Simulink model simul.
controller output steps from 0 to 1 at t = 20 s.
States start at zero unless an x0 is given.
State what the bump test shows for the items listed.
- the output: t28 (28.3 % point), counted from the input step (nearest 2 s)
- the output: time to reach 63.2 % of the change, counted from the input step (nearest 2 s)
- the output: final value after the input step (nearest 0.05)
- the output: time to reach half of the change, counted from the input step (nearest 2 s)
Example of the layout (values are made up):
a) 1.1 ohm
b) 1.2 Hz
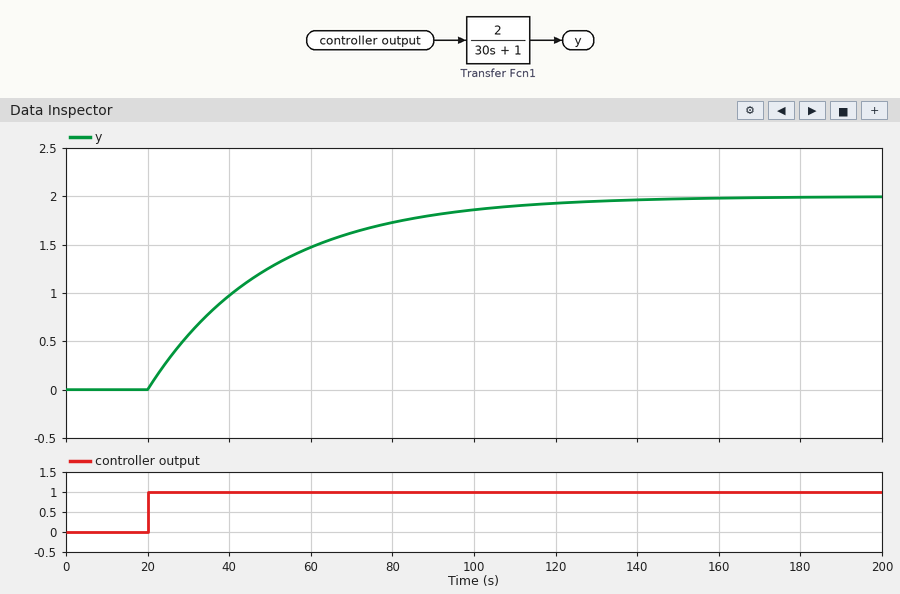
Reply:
a) 10 s
b) 30 s
c) 2.00
d) 20 s
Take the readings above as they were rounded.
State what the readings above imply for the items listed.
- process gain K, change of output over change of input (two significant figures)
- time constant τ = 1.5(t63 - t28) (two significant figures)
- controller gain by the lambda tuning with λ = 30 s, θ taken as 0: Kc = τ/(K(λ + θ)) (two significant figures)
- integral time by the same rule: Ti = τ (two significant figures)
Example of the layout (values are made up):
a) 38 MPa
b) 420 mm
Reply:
a) 2.0
b) 30 s
c) 0.50
d) 30 s
